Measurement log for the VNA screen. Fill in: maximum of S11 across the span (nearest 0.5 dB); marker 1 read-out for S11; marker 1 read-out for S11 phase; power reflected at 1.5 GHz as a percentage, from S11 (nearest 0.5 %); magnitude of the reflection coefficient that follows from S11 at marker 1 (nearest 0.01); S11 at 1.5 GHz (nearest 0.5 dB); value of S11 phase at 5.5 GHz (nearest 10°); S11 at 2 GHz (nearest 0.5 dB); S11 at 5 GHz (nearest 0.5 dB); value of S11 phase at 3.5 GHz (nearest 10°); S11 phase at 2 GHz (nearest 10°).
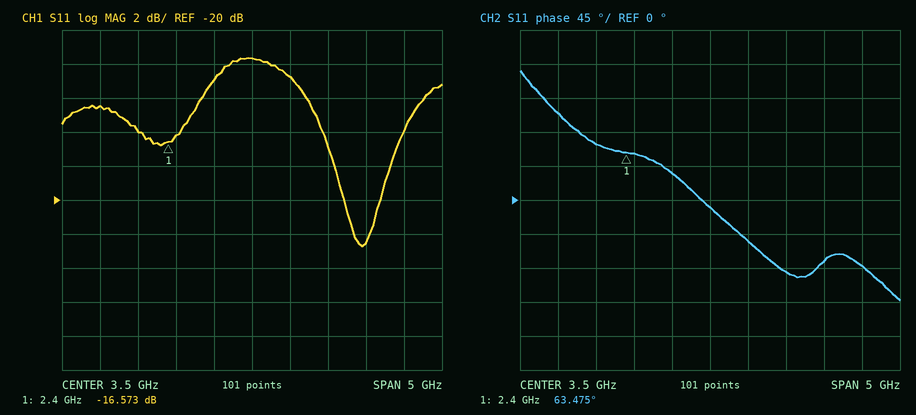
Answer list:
-11.5 dB
-16.573 dB
63.475°
3.5 %
0.15
-14.5 dB
-90°
-16.0 dB
-22.5 dB
-10°
70°
